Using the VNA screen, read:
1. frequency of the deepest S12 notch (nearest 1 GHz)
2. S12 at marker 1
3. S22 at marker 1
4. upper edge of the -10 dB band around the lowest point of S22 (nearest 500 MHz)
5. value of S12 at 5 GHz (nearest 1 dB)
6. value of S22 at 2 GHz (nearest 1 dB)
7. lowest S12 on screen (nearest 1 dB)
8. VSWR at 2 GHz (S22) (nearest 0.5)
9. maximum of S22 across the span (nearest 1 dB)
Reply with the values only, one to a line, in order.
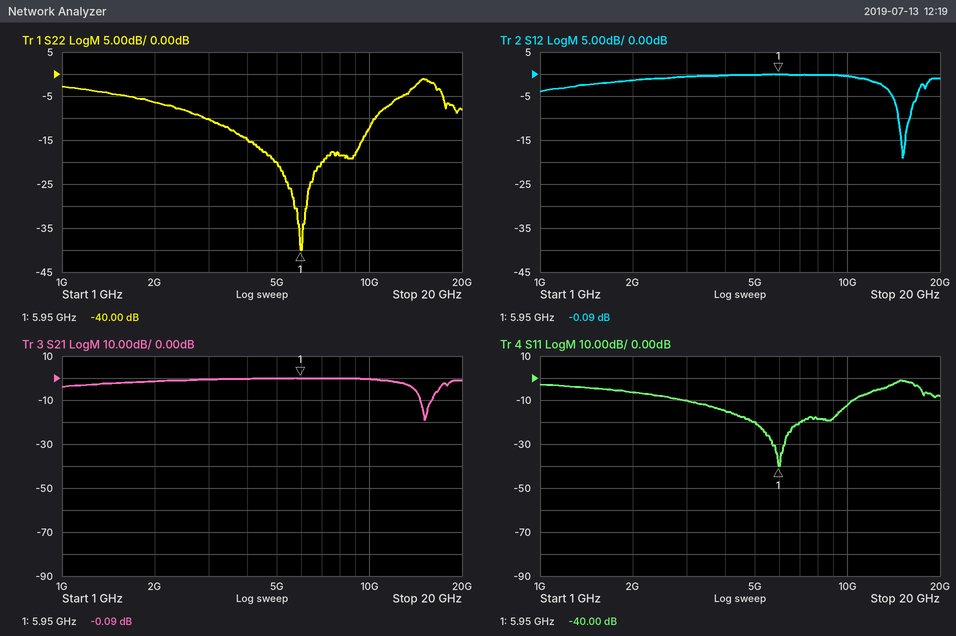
15 GHz
-0.09 dB
-40.00 dB
10.5 GHz
0 dB
-6 dB
-19 dB
3.0
-1 dB
